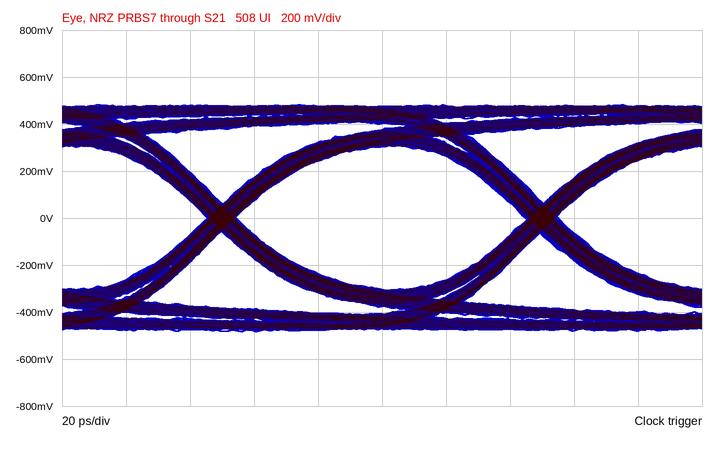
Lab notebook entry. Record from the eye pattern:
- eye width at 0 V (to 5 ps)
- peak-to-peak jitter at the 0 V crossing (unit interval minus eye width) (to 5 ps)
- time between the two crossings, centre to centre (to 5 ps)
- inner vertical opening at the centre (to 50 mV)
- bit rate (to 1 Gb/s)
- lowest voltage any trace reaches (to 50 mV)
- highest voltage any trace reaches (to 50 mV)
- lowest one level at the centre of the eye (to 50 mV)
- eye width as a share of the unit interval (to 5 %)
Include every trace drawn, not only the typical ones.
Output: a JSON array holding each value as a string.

["90 ps", "10 ps", "100 ps", "600 mV", "10 Gb/s", "-500 mV", "500 mV", "300 mV", "90 %"]
